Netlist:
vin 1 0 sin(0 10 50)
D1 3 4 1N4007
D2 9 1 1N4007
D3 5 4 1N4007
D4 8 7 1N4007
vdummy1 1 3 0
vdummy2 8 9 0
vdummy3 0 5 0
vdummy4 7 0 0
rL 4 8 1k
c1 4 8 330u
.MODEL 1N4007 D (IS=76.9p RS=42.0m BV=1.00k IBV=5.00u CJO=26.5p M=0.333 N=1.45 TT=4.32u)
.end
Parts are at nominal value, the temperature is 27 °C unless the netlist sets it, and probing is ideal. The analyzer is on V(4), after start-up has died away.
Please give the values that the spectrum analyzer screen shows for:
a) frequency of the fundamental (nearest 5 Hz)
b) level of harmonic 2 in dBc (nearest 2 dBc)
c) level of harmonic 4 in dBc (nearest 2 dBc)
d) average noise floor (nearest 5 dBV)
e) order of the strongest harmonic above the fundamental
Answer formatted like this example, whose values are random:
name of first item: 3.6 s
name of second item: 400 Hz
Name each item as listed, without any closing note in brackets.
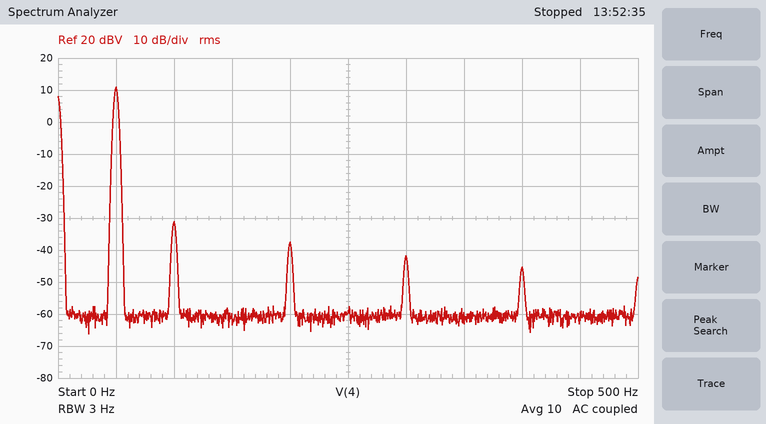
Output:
frequency of the fundamental: 50 Hz
level of harmonic 2 in dBc: -42 dBc
level of harmonic 4 in dBc: -48 dBc
average noise floor: -60 dBV
order of the strongest harmonic above the fundamental: 2
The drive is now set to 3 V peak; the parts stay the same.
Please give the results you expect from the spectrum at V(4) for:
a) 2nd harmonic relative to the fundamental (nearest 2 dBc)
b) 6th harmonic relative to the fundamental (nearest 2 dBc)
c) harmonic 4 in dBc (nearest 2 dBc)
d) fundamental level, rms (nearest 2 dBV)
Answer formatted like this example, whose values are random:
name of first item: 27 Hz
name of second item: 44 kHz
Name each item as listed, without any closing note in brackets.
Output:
2nd harmonic relative to the fundamental: -46 dBc
6th harmonic relative to the fundamental: -60 dBc
harmonic 4 in dBc: -54 dBc
fundamental level, rms: 0 dBV
